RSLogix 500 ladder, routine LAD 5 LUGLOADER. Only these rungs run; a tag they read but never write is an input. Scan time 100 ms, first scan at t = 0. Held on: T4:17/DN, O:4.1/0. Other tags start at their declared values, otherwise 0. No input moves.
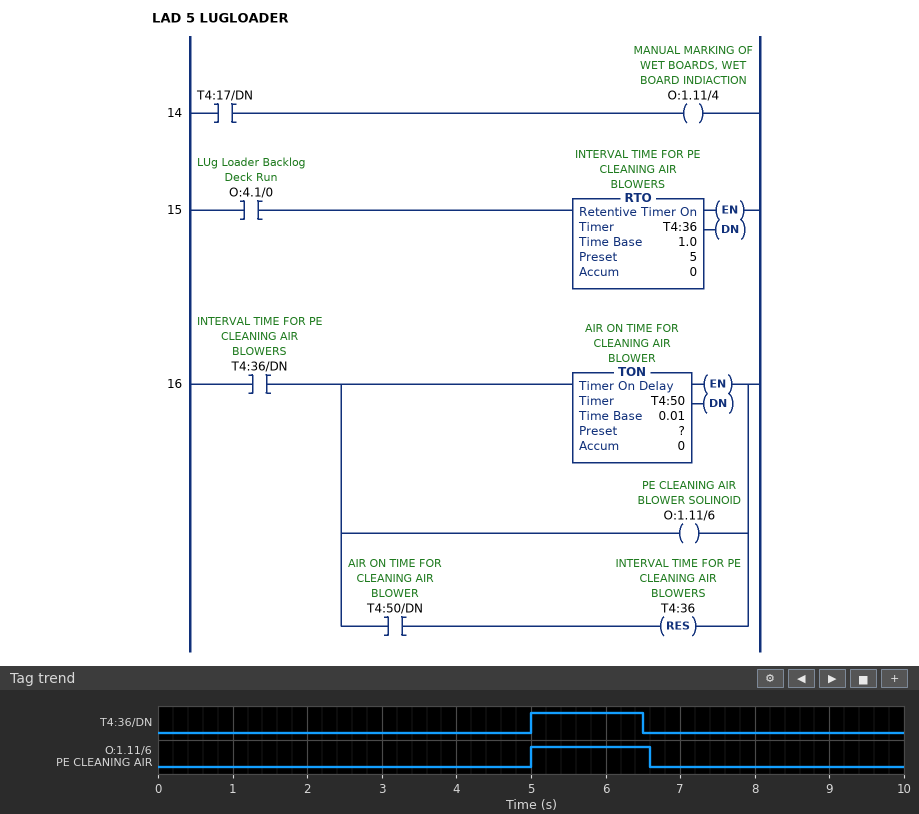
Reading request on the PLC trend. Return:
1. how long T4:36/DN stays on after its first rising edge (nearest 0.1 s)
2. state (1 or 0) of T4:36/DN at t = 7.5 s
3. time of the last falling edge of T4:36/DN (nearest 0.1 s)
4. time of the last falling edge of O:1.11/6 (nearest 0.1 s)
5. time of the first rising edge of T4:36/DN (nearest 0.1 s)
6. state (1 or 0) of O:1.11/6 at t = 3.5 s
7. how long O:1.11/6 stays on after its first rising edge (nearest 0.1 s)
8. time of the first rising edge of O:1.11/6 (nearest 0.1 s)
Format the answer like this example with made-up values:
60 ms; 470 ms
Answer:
1.5 s; 0; 6.5 s; 6.6 s; 5.0 s; 0; 1.6 s; 5.0 s
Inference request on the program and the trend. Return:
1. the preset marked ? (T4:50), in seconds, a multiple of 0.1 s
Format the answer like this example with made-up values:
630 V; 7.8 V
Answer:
1.5 s
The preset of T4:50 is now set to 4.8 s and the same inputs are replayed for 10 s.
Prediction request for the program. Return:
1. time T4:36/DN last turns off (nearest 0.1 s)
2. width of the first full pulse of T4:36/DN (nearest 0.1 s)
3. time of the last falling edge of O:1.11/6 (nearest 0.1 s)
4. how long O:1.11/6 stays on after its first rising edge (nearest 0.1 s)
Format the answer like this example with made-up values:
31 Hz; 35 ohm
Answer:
9.8 s; 4.8 s; 9.9 s; 4.9 s
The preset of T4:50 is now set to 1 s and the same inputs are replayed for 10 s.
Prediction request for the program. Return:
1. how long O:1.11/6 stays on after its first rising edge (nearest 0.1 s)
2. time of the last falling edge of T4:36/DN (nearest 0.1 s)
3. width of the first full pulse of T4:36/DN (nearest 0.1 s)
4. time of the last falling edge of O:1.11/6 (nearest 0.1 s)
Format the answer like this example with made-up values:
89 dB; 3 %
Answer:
1.1 s; 6.0 s; 1.0 s; 6.1 s
